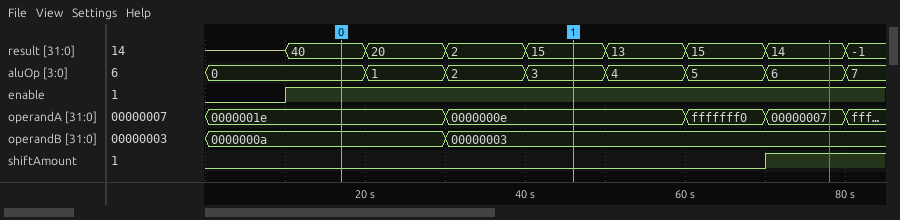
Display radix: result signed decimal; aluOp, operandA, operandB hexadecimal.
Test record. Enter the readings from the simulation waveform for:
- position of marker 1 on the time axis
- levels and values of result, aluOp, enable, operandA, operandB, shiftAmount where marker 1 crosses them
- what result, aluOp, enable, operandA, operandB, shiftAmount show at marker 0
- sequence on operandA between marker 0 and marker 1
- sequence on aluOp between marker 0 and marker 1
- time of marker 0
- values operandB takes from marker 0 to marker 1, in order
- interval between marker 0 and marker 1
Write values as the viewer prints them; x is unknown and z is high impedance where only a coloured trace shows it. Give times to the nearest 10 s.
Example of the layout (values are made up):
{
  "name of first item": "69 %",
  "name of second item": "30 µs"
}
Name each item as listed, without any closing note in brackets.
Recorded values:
{
  "position of marker 1 on the time axis": "50 s",
  "levels and values of result, aluOp, enable, operandA, operandB, shiftAmount where marker 1 crosses them": "result=15, aluOp=3, enable=1, operandA=0000000e, operandB=00000003, shiftAmount=0",
  "what result, aluOp, enable, operandA, operandB, shiftAmount show at marker 0": "result=40, aluOp=0, enable=1, operandA=0000001e, operandB=0000000a, shiftAmount=0",
  "sequence on operandA between marker 0 and marker 1": "0000001e, 0000000e",
  "sequence on aluOp between marker 0 and marker 1": "0, 1, 2, 3",
  "time of marker 0": "20 s",
  "values operandB takes from marker 0 to marker 1, in order": "0000000a, 00000003",
  "interval between marker 0 and marker 1": "30 s"
}
